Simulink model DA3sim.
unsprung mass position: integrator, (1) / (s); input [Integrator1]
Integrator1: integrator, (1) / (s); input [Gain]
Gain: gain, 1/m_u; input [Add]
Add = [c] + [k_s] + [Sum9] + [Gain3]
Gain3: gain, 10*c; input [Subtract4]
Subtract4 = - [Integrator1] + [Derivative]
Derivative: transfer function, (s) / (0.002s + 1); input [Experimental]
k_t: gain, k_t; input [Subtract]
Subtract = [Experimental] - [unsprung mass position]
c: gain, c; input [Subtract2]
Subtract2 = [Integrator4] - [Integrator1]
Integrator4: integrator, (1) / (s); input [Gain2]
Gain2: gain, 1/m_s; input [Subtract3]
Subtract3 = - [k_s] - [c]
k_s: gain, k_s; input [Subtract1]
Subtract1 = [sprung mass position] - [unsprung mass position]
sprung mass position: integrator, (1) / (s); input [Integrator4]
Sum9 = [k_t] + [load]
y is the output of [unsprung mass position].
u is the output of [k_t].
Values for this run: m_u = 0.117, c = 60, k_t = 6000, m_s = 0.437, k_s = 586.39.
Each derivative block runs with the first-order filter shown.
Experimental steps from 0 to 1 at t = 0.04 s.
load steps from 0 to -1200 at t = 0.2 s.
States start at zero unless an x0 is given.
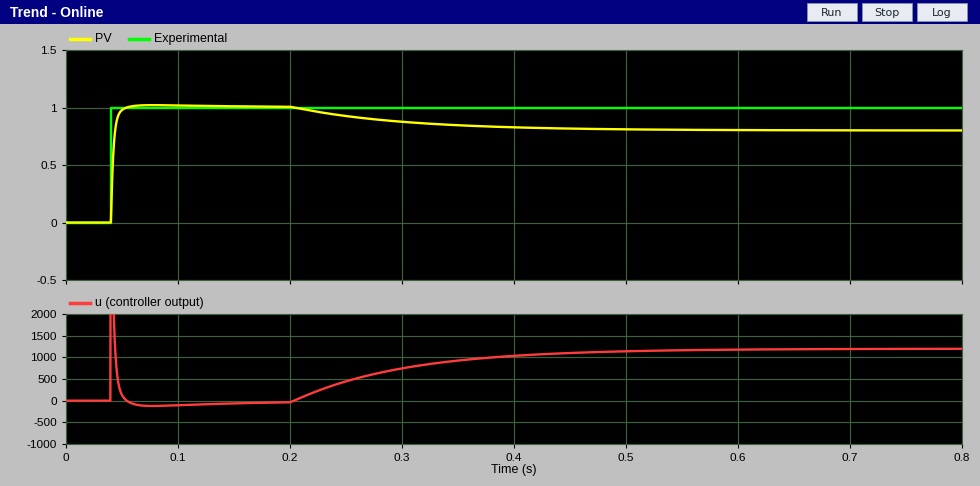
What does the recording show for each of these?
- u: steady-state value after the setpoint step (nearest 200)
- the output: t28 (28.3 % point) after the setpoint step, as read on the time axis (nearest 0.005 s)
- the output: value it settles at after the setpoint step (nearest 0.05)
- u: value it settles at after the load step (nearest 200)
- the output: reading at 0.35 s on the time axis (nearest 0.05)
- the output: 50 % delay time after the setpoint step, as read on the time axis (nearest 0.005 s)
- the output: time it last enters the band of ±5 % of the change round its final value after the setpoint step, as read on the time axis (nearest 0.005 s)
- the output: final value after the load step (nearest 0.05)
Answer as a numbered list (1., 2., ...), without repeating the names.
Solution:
1. 0
2. 0.040 s
3. 1.00
4. 1200
5. 0.85
6. 0.040 s
7. 0.050 s
8. 0.80
